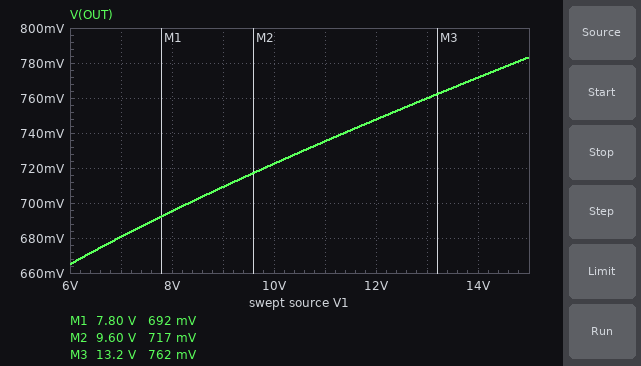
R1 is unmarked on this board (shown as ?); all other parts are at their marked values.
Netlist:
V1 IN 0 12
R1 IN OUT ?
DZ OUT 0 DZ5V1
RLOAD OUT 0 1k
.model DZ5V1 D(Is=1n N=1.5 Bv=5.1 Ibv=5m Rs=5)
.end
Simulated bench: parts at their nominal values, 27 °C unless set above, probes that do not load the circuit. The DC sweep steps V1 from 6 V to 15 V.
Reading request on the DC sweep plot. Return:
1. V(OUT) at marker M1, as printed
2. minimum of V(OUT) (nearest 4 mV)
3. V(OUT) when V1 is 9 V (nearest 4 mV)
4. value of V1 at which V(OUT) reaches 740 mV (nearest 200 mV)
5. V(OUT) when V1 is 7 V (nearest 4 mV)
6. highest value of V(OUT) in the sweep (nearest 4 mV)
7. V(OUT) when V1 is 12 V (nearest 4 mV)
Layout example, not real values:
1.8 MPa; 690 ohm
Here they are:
692 mV; 664 mV; 708 mV; 11.4 V; 680 mV; 784 mV; 748 mV
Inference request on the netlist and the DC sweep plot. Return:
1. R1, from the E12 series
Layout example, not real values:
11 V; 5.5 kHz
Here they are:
560 Ω
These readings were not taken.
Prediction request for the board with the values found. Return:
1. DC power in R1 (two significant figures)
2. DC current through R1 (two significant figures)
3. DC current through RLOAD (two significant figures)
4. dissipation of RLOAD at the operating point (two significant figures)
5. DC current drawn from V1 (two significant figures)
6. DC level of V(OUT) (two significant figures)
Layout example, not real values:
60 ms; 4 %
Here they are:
230 mW; 20 mA; 750 µA; 560 µW; 20 mA; 750 mV
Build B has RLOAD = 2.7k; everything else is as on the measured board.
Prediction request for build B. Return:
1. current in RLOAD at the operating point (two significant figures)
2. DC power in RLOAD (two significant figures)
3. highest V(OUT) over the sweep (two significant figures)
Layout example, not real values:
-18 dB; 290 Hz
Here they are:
280 µA; 210 µW; 790 mV
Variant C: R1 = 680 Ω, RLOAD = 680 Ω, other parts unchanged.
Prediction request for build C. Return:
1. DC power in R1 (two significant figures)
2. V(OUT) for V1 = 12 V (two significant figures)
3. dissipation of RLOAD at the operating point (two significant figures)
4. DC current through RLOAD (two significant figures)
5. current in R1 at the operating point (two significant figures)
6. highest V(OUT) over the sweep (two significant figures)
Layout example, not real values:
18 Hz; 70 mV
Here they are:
190 mW; 720 mV; 760 µW; 1.1 mA; 17 mA; 750 mV
